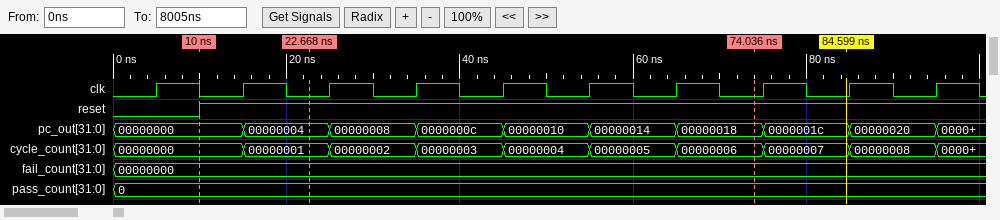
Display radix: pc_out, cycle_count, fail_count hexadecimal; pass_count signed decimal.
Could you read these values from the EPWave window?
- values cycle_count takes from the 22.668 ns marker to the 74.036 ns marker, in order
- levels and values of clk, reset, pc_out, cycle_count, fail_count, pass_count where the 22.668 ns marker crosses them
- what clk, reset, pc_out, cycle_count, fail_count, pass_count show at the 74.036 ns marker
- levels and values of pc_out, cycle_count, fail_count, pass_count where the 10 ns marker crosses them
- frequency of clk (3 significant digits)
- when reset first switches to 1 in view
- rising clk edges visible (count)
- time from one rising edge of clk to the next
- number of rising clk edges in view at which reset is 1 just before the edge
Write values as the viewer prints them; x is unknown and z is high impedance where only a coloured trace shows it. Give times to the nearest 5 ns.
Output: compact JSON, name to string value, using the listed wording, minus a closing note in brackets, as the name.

{"values cycle_count takes from the 22.668 ns marker to the 74.036 ns marker, in order": "00000001, 00000002, 00000003, 00000004, 00000005, 00000006", "levels and values of clk, reset, pc_out, cycle_count, fail_count, pass_count where the 22.668 ns marker crosses them": "clk=0, reset=1, pc_out=00000004, cycle_count=00000001, fail_count=00000000, pass_count=0", "what clk, reset, pc_out, cycle_count, fail_count, pass_count show at the 74.036 ns marker": "clk=0, reset=1, pc_out=00000018, cycle_count=00000006, fail_count=00000000, pass_count=0", "levels and values of pc_out, cycle_count, fail_count, pass_count where the 10 ns marker crosses them": "pc_out=00000000, cycle_count=00000000, fail_count=00000000, pass_count=0", "frequency of clk": "100 MHz", "when reset first switches to 1 in view": "10 ns", "rising clk edges visible": "10", "time from one rising edge of clk to the next": "10 ns", "number of rising clk edges in view at which reset is 1 just before the edge": "9"}
